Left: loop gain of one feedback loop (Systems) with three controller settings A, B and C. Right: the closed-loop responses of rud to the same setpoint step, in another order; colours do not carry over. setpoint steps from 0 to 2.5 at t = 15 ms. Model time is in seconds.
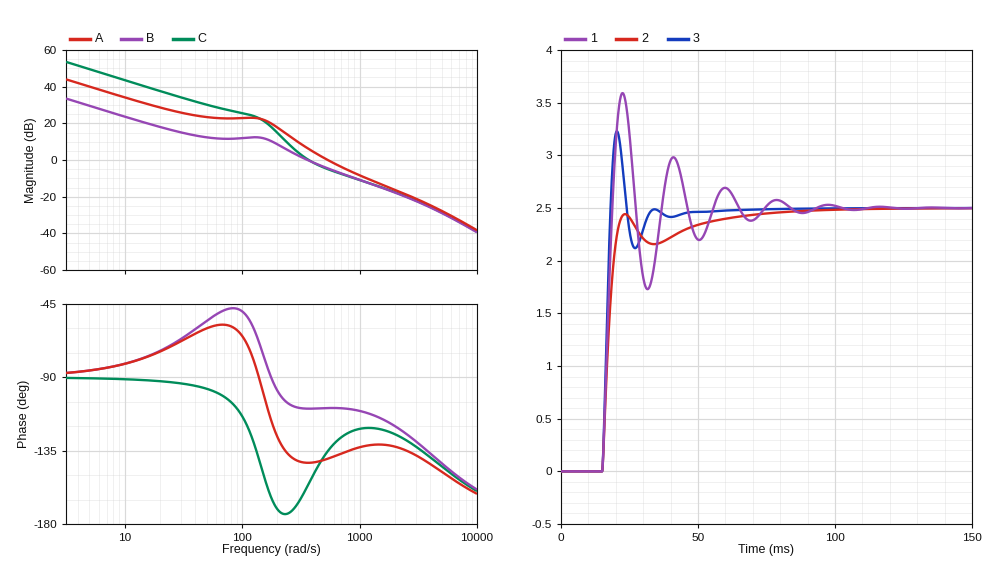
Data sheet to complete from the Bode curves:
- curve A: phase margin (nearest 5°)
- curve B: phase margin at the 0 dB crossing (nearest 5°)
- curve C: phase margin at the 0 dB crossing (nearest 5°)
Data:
40°
70°
25°
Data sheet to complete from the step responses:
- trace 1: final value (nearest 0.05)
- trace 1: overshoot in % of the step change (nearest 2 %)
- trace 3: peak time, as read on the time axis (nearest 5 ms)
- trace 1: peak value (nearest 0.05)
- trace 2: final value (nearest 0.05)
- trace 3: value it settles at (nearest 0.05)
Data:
2.50
44 %
20 ms
3.60
2.50
2.50
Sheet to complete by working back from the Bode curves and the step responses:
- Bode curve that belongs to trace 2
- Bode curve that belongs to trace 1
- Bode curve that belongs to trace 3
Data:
B
C
A
